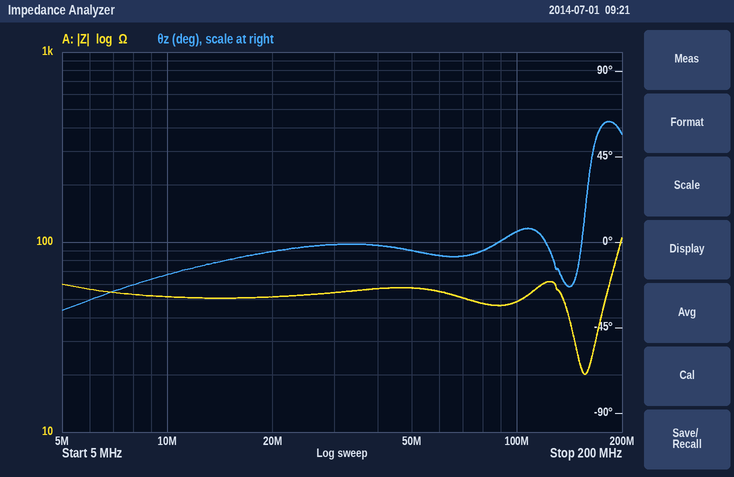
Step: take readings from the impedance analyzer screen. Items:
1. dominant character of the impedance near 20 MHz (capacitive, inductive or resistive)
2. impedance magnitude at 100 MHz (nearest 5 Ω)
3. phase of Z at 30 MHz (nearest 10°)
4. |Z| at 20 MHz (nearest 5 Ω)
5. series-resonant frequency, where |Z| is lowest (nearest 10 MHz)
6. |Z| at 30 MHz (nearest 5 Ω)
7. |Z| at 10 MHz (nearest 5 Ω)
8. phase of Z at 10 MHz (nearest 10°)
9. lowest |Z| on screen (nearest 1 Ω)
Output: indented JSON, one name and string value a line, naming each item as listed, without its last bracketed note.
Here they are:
{
  "dominant character of the impedance near 20 MHz": "resistive",
  "impedance magnitude at 100 MHz": "50 Ω",
  "phase of Z at 30 MHz": "0°",
  "|Z| at 20 MHz": "50 Ω",
  "series-resonant frequency, where |Z| is lowest": "160 MHz",
  "|Z| at 30 MHz": "55 Ω",
  "|Z| at 10 MHz": "50 Ω",
  "phase of Z at 10 MHz": "-20°",
  "lowest |Z| on screen": "20 Ω"
}
